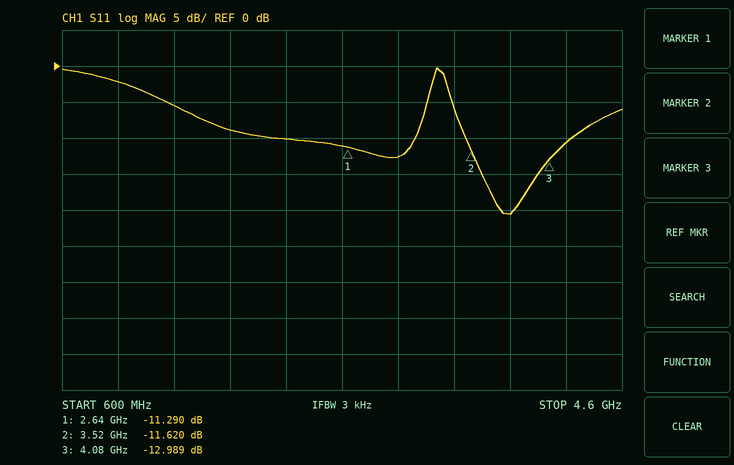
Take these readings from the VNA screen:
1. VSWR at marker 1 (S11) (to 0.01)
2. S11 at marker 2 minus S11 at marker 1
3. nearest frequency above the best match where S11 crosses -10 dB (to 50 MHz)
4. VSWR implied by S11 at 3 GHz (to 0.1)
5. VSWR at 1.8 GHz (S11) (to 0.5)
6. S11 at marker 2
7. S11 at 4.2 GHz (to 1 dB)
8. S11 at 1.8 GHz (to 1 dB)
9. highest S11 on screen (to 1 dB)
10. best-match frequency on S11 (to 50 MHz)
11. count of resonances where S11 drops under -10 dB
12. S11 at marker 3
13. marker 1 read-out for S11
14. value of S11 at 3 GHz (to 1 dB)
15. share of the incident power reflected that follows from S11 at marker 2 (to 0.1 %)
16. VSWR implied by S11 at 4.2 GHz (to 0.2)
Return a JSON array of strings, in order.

["1.75", "-0.330 dB", "4.25 GHz", "1.6", "2.0", "-11.620 dB", "-11 dB", "-9 dB", "0 dB", "3.80 GHz", "2", "-12.989 dB", "-11.290 dB", "-13 dB", "6.9 %", "1.8"]
